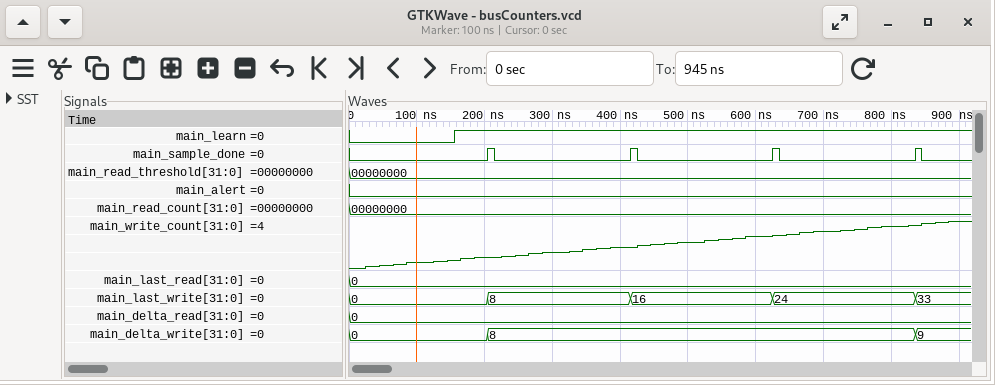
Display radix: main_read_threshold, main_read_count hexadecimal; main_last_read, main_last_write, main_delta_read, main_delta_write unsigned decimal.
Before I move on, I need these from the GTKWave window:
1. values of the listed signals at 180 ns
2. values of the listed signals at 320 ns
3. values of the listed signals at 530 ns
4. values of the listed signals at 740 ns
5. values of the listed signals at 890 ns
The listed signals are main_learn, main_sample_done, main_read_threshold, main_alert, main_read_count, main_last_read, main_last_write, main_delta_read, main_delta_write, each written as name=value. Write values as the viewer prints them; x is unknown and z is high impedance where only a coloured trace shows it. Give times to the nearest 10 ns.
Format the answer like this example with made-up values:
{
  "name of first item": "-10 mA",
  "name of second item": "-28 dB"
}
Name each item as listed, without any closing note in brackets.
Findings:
{
  "values of the listed signals at 180 ns": "main_learn=1, main_sample_done=0, main_read_threshold=00000000, main_alert=0, main_read_count=00000000, main_last_read=0, main_last_write=0, main_delta_read=0, main_delta_write=0",
  "values of the listed signals at 320 ns": "main_learn=1, main_sample_done=0, main_read_threshold=00000000, main_alert=0, main_read_count=00000000, main_last_read=0, main_last_write=8, main_delta_read=0, main_delta_write=8",
  "values of the listed signals at 530 ns": "main_learn=1, main_sample_done=0, main_read_threshold=00000000, main_alert=0, main_read_count=00000000, main_last_read=0, main_last_write=16, main_delta_read=0, main_delta_write=8",
  "values of the listed signals at 740 ns": "main_learn=1, main_sample_done=0, main_read_threshold=00000000, main_alert=0, main_read_count=00000000, main_last_read=0, main_last_write=24, main_delta_read=0, main_delta_write=8",
  "values of the listed signals at 890 ns": "main_learn=1, main_sample_done=0, main_read_threshold=00000000, main_alert=0, main_read_count=00000000, main_last_read=0, main_last_write=33, main_delta_read=0, main_delta_write=9"
}
